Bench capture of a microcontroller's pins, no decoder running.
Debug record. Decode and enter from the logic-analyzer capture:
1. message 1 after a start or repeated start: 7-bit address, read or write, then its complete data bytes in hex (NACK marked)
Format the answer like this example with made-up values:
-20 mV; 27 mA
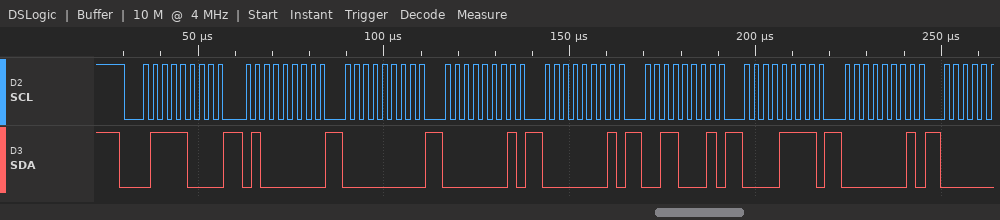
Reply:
0x3C write: 40 00 01 01 31 0F 01
